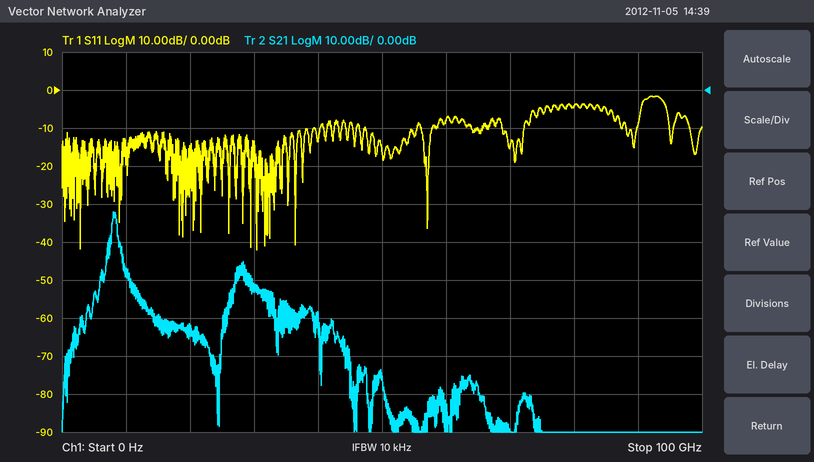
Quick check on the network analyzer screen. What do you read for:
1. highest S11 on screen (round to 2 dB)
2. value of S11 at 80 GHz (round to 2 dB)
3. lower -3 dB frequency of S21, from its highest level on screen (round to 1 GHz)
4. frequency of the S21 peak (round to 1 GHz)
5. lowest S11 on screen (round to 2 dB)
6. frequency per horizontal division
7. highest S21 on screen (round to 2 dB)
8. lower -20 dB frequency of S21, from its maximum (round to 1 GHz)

-2 dB
-4 dB
8 GHz
8 GHz
-42 dB
10 GHz
-32 dB
6 GHz
